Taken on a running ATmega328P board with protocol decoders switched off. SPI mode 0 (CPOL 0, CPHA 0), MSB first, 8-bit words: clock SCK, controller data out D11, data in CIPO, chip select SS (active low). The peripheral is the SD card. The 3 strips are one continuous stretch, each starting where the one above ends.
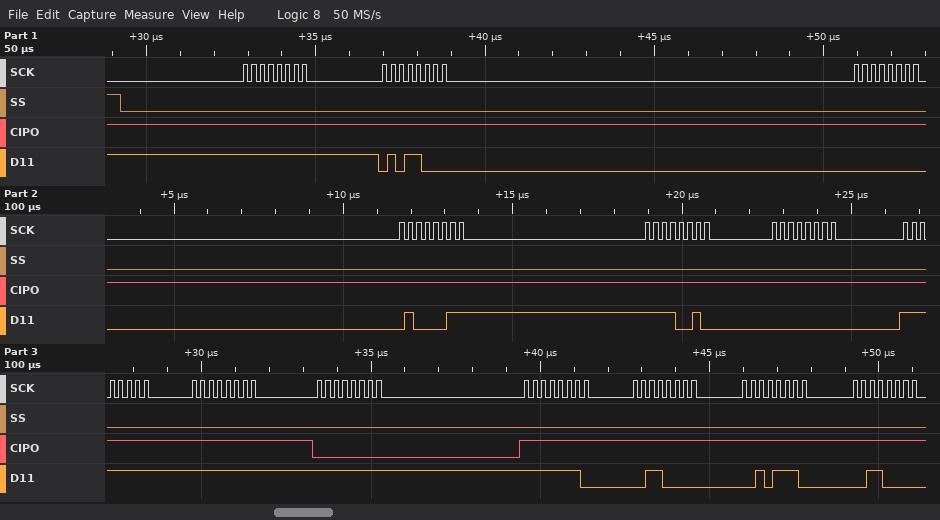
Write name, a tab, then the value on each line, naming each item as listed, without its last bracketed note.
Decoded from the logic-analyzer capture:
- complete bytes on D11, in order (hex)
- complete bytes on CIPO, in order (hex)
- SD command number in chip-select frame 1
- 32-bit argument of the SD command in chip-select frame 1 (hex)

complete bytes on D11, in order	FF 58 00 43 F2 00 FF FF FF FE 30 2E 30
complete bytes on CIPO, in order	FF FF FF FF FF FF FF FF 00 FF FF FF FF
SD command number in chip-select frame 1	CMD24
32-bit argument of the SD command in chip-select frame 1	0x0043F200
